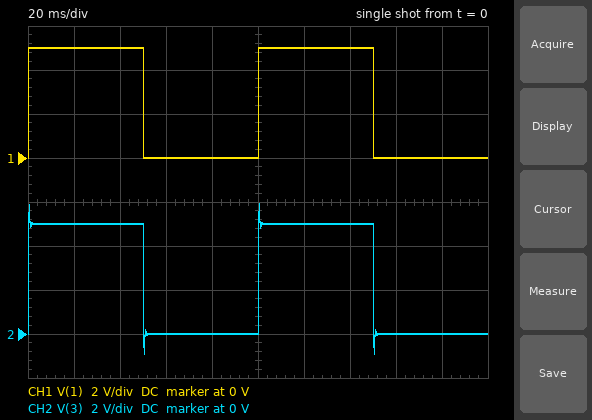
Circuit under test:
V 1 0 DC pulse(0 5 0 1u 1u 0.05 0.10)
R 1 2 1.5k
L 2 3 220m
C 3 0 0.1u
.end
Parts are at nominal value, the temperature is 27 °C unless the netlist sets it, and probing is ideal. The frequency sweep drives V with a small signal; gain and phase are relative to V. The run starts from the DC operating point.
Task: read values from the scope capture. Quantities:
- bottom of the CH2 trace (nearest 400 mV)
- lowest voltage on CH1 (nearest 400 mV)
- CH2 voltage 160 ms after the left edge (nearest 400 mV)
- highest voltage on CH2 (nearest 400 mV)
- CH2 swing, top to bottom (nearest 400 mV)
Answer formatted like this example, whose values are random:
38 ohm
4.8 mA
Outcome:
-800 mV
0 V
0 V
6.0 V
6.8 V
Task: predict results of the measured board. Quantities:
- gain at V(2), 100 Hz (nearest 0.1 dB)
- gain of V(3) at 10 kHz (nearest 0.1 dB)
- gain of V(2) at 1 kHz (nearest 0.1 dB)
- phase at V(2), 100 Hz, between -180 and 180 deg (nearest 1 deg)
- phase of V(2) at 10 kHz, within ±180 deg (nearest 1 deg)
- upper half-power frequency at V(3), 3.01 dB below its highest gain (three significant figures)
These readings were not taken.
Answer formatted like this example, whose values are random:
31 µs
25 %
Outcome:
0 dB
-38.7 dB
-17.2 dB
-5 deg
6 deg
1.25 kHz
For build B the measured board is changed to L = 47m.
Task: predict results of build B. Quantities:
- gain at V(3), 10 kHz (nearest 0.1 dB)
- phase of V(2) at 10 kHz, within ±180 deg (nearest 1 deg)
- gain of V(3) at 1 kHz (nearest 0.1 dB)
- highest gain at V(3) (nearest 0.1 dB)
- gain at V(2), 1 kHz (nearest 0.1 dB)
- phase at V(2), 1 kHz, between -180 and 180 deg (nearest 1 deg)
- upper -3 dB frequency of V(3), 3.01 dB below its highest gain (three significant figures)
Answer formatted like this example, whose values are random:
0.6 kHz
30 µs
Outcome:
-26.0 dB
28 deg
-1.9 dB
0 dB
-3.7 dB
-49 deg
1.32 kHz
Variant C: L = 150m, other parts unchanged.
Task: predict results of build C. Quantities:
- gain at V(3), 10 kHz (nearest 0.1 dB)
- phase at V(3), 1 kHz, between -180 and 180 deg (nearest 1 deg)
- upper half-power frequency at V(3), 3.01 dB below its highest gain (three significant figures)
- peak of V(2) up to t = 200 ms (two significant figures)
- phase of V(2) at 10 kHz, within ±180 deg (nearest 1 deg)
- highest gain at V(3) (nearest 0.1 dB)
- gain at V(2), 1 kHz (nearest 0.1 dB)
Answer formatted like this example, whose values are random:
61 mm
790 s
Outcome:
-35.4 dB
-67 deg
1.43 kHz
5.3 V
9 deg
0.3 dB
-8.0 dB
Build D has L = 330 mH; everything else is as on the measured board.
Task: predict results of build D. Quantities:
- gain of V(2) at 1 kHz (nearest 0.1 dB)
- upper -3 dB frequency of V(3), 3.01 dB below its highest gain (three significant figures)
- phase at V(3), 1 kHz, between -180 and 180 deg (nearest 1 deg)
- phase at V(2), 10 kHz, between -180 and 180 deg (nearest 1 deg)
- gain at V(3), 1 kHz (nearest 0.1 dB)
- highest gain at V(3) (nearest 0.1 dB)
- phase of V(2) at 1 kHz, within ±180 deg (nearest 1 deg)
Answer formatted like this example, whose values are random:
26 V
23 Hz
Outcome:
-10.3 dB
1.04 kHz
-108 deg
4 deg
0.1 dB
2.5 dB
72 deg
